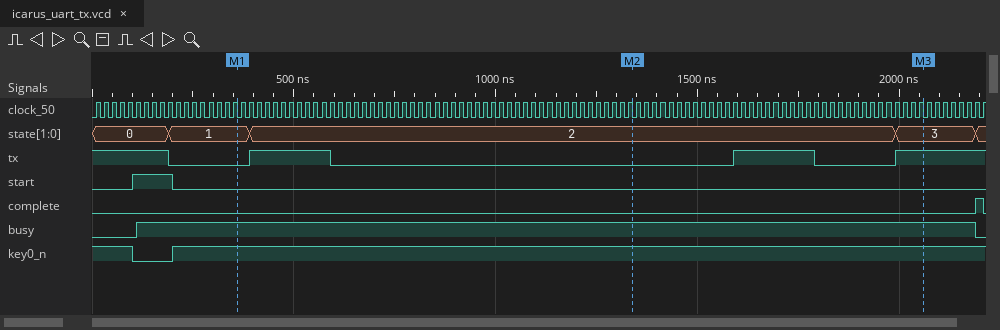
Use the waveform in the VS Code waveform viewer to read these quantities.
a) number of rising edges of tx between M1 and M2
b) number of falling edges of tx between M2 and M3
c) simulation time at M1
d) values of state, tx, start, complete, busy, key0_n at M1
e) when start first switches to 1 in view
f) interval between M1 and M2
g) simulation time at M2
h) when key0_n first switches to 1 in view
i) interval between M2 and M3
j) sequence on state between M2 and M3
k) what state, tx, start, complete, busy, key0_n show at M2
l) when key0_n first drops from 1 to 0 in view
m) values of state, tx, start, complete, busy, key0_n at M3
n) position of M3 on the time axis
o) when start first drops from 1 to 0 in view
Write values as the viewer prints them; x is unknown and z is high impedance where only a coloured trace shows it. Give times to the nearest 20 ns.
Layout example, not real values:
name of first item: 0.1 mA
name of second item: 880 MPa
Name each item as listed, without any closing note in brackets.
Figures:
number of rising edges of tx between M1 and M2: 1
number of falling edges of tx between M2 and M3: 1
simulation time at M1: 360 ns
values of state, tx, start, complete, busy, key0_n at M1: state=1, tx=0, start=0, complete=0, busy=1, key0_n=1
when start first switches to 1 in view: 100 ns
interval between M1 and M2: 980 ns
simulation time at M2: 1340 ns
when key0_n first switches to 1 in view: 200 ns
interval between M2 and M3: 720 ns
sequence on state between M2 and M3: 2, 3
what state, tx, start, complete, busy, key0_n show at M2: state=2, tx=0, start=0, complete=0, busy=1, key0_n=1
when key0_n first drops from 1 to 0 in view: 100 ns
values of state, tx, start, complete, busy, key0_n at M3: state=3, tx=1, start=0, complete=0, busy=1, key0_n=1
position of M3 on the time axis: 2060 ns
when start first drops from 1 to 0 in view: 200 ns
